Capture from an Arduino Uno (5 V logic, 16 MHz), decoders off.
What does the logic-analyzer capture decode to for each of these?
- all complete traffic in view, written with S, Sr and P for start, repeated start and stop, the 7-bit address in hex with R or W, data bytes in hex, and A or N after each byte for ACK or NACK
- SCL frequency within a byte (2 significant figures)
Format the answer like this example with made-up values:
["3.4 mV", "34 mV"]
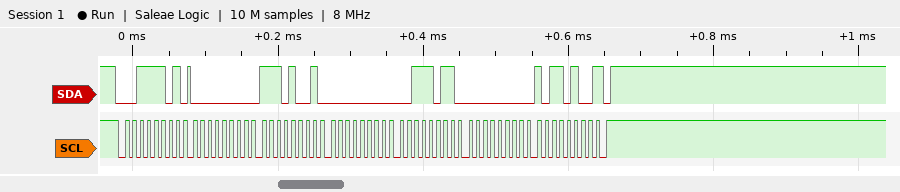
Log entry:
["S 1ER A 00 A E9 A 00 A 3B A 00 A B4 N P", "100 kHz"]
